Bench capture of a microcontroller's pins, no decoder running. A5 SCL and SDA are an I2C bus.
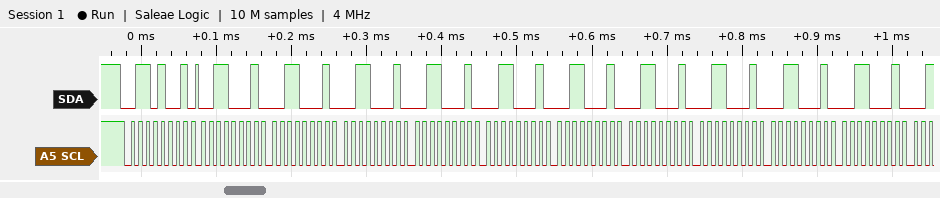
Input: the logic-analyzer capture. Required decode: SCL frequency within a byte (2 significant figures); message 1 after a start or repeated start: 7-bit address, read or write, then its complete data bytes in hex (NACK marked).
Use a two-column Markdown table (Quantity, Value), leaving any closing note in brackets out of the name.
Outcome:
| Quantity | Value |
|---|---|
| SCL frequency within a byte | 100 kHz |
| message 1 after a start or repeated start: 7-bit address, read or write, then its complete data bytes in hex | 0x34 read: 31 31 31 31 31 31 31 31 31 31 |
